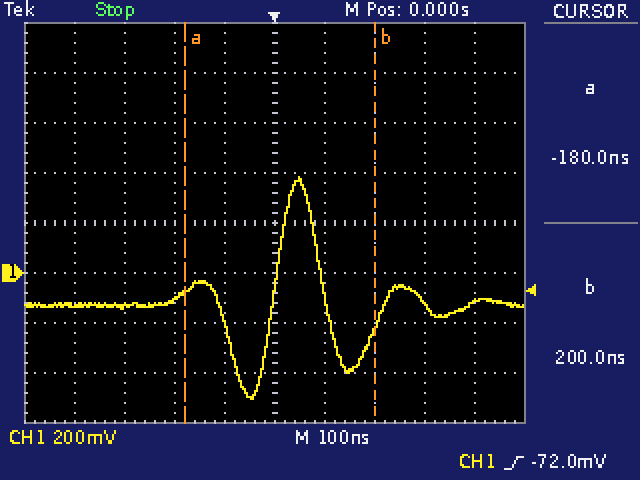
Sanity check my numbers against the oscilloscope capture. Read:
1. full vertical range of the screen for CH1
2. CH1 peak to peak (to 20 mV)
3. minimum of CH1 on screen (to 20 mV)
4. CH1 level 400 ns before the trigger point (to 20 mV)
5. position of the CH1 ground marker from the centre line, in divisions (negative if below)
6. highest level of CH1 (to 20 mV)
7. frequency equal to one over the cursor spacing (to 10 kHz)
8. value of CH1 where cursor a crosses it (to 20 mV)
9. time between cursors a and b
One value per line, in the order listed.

1.6 V
880 mV
-500 mV
-120 mV
-1.0 div
380 mV
2.63 MHz
-80 mV
380 ns
